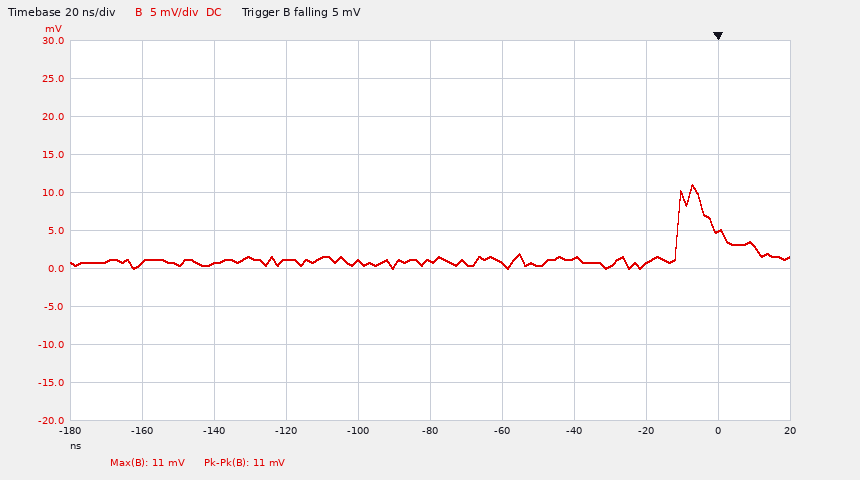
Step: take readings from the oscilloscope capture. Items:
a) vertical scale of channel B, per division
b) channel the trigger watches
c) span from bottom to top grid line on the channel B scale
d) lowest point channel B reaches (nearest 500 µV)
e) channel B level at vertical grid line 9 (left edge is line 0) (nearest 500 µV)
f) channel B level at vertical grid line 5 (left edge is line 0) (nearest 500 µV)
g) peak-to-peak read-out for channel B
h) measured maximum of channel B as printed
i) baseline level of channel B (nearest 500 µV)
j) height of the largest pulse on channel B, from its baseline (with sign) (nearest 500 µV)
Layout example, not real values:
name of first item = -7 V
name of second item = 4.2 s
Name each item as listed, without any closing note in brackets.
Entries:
vertical scale of channel B, per division = 5 mV
channel the trigger watches = channel B
span from bottom to top grid line on the channel B scale = 50 mV
lowest point channel B reaches = 0.0 mV
channel B level at vertical grid line 9 (left edge is line 0) = 5.0 mV
channel B level at vertical grid line 5 (left edge is line 0) = 1.0 mV
peak-to-peak read-out for channel B = 11 mV
measured maximum of channel B as printed = 11 mV
baseline level of channel B = 1.0 mV
height of the largest pulse on channel B, from its baseline (with sign) = +10.0 mV
